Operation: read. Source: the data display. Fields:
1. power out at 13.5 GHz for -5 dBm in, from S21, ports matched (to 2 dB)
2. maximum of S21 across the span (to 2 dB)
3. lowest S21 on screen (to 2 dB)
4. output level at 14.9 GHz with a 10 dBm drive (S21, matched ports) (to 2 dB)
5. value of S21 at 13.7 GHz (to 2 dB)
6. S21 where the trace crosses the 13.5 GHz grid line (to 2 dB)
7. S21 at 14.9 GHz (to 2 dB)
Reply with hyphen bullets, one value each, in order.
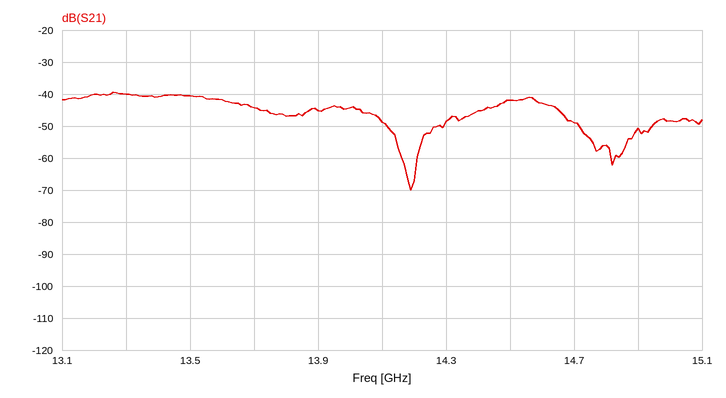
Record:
- -46 dBm
- -40 dB
- -70 dB
- -40 dBm
- -44 dB
- -40 dB
- -50 dB
